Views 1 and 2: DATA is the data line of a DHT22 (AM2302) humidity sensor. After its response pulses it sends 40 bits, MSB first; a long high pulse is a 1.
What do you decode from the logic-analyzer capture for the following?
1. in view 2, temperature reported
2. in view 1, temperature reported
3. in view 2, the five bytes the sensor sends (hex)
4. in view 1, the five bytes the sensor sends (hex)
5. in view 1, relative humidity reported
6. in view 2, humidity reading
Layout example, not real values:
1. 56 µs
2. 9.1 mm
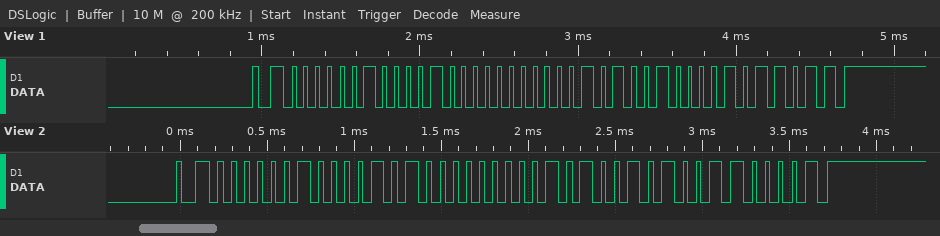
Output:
1. 33.0 °C
2. 32.8 °C
3. 02 14 01 4A 61
4. 02 10 01 48 5B
5. 52.8 %
6. 53.2 %
